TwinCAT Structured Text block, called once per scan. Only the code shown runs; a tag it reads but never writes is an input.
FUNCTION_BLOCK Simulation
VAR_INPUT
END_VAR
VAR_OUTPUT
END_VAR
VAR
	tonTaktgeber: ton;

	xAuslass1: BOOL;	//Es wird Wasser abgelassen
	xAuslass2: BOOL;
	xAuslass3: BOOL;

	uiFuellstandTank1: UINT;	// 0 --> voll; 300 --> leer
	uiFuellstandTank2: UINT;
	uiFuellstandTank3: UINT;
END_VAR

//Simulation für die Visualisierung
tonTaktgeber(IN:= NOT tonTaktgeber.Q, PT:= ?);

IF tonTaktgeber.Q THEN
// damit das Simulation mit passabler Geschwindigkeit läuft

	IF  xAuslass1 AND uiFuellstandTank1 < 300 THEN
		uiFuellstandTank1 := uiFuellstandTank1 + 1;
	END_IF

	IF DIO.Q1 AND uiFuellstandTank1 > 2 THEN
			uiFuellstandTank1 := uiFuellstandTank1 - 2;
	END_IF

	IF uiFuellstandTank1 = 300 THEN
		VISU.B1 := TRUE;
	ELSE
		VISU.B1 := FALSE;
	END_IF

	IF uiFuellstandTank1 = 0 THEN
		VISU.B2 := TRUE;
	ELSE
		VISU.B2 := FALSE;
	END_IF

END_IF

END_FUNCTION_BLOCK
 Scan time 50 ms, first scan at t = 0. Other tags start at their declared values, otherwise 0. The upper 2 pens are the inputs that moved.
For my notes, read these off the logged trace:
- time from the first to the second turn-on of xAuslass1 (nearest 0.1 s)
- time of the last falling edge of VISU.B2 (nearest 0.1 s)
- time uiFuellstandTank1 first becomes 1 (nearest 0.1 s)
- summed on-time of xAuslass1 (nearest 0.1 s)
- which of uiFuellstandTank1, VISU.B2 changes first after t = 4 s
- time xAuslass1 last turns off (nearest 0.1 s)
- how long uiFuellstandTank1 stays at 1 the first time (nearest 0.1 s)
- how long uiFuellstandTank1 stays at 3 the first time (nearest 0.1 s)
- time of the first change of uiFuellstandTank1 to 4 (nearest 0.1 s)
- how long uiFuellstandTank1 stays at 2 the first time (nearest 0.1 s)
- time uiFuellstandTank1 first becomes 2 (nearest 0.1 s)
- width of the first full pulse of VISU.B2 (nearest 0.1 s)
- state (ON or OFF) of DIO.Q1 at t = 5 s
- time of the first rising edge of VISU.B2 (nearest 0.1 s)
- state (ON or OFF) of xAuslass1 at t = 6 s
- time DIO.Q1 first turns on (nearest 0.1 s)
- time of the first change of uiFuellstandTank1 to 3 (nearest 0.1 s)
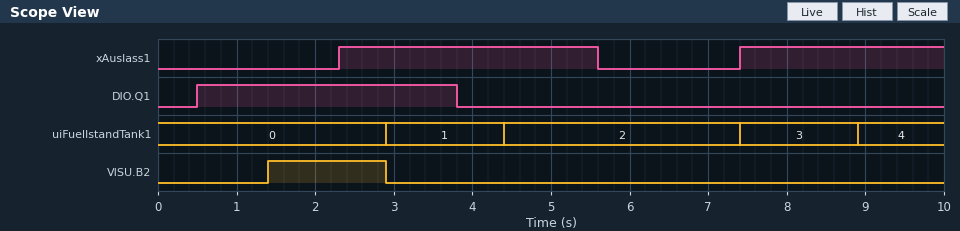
5.1 s
2.9 s
2.9 s
5.9 s
uiFuellstandTank1
5.6 s
1.5 s
1.5 s
8.9 s
3.0 s
4.4 s
1.5 s
OFF
1.4 s
OFF
0.5 s
7.4 s
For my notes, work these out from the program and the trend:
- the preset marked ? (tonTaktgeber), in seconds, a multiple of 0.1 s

1.4 s
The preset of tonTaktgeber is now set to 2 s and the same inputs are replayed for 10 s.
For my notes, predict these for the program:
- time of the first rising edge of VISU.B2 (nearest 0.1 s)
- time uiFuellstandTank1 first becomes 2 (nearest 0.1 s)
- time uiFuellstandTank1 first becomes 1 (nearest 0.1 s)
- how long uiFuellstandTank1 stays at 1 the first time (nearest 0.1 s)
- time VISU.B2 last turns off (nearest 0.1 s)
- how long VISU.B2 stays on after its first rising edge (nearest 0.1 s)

2.0 s
8.3 s
4.1 s
4.2 s
4.1 s
2.1 s
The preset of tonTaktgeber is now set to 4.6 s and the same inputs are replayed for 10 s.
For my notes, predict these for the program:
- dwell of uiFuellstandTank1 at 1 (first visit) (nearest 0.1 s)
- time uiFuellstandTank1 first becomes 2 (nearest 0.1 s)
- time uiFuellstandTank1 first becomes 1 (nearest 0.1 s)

4.7 s
9.3 s
4.6 s
